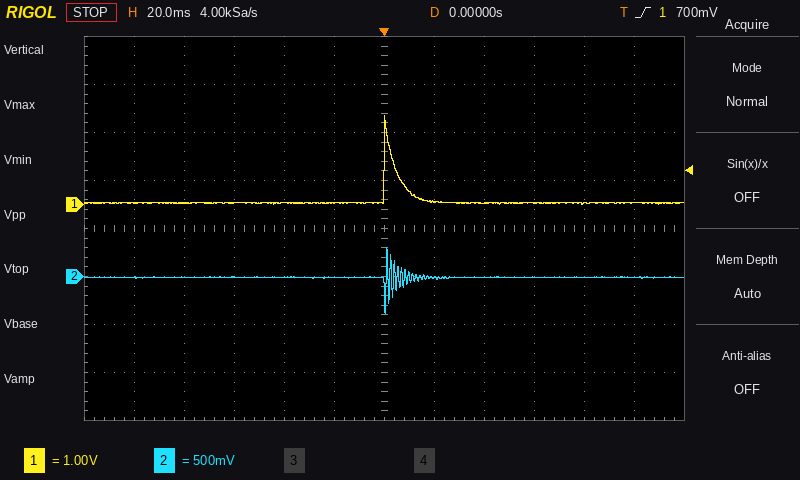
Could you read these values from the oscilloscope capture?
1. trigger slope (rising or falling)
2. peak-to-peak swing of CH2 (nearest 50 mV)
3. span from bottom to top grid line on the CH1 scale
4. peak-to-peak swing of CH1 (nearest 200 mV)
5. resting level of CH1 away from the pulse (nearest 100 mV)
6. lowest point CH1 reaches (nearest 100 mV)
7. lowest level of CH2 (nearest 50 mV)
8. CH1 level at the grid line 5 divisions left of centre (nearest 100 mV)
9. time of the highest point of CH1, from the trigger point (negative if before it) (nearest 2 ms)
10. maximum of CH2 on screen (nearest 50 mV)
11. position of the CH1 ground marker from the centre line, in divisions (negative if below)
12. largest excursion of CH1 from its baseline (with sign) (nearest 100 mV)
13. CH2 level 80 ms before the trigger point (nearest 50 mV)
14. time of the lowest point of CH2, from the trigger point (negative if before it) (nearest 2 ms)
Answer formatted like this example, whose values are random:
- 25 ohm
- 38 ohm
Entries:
- rising
- 700 mV
- 8 V
- 1.8 V
- 0.0 V
- 0.0 V
- -400 mV
- 0.0 V
- 0 ms
- 300 mV
- +0.5 div
- +1.8 V
- 0 mV
- 0 ms
